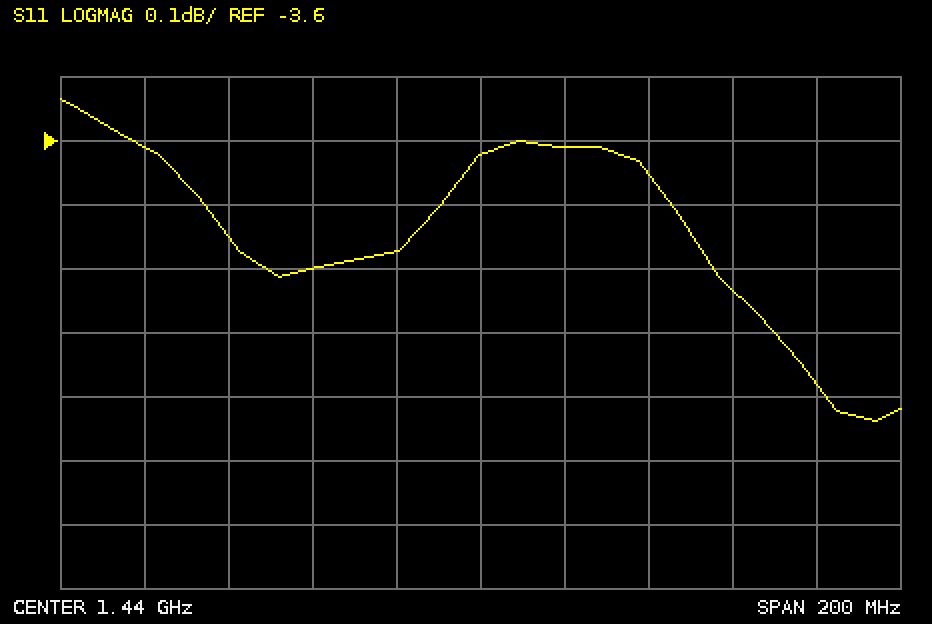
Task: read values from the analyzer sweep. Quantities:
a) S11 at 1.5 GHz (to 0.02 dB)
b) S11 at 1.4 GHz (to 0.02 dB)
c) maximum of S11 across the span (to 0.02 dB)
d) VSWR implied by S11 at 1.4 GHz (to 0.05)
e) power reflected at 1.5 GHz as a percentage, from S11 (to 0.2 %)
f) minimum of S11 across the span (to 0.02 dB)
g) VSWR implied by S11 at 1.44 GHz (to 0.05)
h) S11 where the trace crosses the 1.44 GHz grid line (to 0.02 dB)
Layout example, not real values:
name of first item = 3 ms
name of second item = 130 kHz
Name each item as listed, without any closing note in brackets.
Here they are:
S11 at 1.5 GHz = -3.84 dB
S11 at 1.4 GHz = -3.80 dB
maximum of S11 across the span = -3.54 dB
VSWR implied by S11 at 1.4 GHz = 4.65
power reflected at 1.5 GHz as a percentage, from S11 = 41.4 %
minimum of S11 across the span = -4.04 dB
VSWR implied by S11 at 1.44 GHz = 4.85
S11 where the trace crosses the 1.44 GHz grid line = -3.62 dB
